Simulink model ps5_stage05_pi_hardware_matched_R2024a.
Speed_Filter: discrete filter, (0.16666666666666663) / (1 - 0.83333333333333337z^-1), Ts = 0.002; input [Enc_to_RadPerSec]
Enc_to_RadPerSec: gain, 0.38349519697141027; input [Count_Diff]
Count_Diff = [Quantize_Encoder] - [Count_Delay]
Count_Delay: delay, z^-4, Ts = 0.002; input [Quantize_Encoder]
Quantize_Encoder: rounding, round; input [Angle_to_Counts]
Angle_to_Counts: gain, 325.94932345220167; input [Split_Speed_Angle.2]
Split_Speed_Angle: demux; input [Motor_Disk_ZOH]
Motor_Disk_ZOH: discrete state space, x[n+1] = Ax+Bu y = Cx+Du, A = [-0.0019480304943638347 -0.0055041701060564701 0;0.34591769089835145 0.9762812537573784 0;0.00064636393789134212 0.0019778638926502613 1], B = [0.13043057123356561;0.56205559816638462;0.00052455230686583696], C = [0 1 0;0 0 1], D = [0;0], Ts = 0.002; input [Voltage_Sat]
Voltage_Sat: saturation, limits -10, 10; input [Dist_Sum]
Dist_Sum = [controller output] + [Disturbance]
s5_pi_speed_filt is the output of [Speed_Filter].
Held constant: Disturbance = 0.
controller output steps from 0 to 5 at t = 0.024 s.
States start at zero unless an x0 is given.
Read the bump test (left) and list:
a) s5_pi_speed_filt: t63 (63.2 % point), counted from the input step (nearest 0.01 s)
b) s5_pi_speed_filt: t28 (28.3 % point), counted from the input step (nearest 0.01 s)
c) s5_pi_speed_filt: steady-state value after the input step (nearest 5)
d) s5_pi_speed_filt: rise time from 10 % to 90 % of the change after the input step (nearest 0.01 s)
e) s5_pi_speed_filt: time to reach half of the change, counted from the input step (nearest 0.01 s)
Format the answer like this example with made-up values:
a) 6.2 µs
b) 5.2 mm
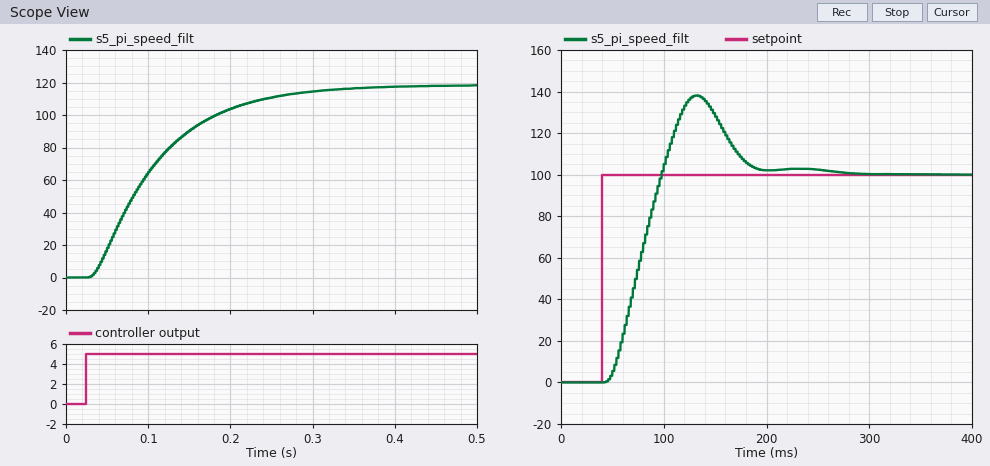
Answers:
a) 0.09 s
b) 0.04 s
c) 120
d) 0.17 s
e) 0.07 s
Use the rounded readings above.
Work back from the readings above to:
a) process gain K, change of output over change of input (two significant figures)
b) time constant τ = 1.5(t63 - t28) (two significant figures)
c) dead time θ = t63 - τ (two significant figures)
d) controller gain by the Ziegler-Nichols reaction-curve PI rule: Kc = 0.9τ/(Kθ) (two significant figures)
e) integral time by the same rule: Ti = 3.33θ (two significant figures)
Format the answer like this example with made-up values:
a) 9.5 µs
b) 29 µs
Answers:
a) 24
b) 0.075 s
c) 0.015 s
d) 0.19
e) 0.050 s
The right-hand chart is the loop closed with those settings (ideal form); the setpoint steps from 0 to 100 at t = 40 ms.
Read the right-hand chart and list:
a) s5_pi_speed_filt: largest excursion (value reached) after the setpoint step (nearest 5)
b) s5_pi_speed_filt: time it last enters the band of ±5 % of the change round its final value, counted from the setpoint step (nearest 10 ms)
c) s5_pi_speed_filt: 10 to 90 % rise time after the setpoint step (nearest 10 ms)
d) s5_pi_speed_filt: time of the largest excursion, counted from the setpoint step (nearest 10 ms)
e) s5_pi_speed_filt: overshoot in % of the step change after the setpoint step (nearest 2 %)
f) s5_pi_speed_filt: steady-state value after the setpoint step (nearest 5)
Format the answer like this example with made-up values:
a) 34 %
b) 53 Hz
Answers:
a) 140
b) 140 ms
c) 40 ms
d) 90 ms
e) 38 %
f) 100
